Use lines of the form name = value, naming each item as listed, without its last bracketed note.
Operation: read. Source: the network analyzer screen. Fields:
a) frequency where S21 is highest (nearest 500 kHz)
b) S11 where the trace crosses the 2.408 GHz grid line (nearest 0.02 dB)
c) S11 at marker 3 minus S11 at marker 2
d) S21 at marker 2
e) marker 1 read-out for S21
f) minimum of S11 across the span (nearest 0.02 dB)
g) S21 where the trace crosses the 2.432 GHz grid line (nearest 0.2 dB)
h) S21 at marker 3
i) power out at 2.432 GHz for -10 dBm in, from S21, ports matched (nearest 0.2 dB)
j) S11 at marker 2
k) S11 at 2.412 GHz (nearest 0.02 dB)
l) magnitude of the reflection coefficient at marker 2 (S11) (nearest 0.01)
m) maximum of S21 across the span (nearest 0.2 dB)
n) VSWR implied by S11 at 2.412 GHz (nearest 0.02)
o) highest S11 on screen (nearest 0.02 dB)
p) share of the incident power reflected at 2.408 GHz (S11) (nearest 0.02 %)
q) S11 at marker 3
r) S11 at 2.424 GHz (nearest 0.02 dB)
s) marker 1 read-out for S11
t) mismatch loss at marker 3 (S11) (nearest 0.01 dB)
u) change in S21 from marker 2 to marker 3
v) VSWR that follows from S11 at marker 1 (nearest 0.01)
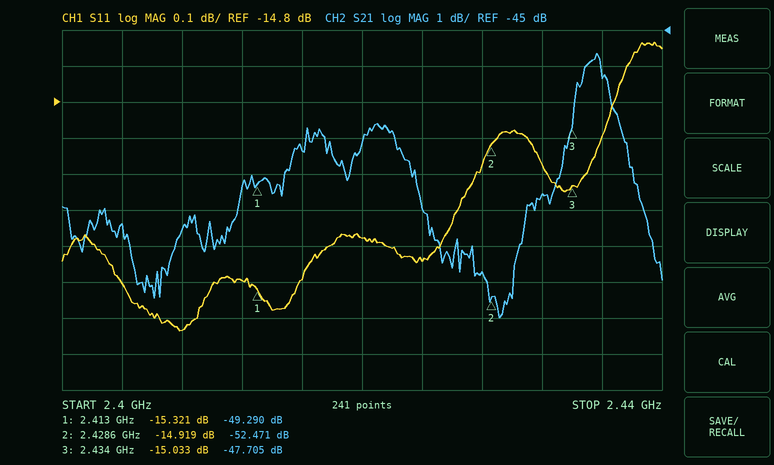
frequency where S21 is highest = 2.4355 GHz
S11 where the trace crosses the 2.408 GHz grid line = -15.44 dB
S11 at marker 3 minus S11 at marker 2 = -0.114 dB
S21 at marker 2 = -52.471 dB
marker 1 read-out for S21 = -49.290 dB
minimum of S11 across the span = -15.44 dB
S21 where the trace crosses the 2.432 GHz grid line = -49.6 dB
S21 at marker 3 = -47.705 dB
power out at 2.432 GHz for -10 dBm in, from S21, ports matched = -59.6 dBm
S11 at marker 2 = -14.919 dB
S11 at 2.412 GHz = -15.30 dB
magnitude of the reflection coefficient at marker 2 (S11) = 0.18
maximum of S21 across the span = -45.6 dB
VSWR implied by S11 at 2.412 GHz = 1.42
highest S11 on screen = -14.64 dB
share of the incident power reflected at 2.408 GHz (S11) = 2.86 %
S11 at marker 3 = -15.033 dB
S11 at 2.424 GHz = -15.24 dB
marker 1 read-out for S11 = -15.321 dB
mismatch loss at marker 3 (S11) = 0.14 dB
change in S21 from marker 2 to marker 3 = 4.766 dB
VSWR that follows from S11 at marker 1 = 1.41
